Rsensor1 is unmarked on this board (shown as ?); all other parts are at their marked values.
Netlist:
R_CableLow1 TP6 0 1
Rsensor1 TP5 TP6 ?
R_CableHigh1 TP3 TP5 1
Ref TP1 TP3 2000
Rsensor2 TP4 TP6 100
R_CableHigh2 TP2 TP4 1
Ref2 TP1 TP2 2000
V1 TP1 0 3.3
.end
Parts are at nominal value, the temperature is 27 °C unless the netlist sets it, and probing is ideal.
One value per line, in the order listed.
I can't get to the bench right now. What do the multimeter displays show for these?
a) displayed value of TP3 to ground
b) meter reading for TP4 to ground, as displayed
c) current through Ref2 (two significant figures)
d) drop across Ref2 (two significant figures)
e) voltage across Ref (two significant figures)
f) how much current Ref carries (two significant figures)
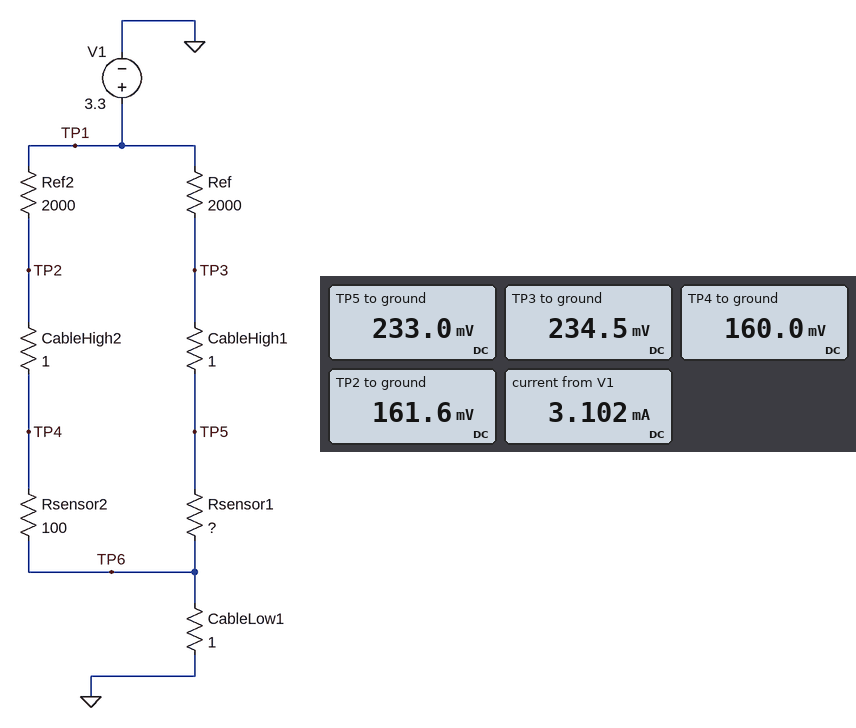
234.5 mV
160.0 mV
1.6 mA
3.1 V
3.1 V
1.5 mA
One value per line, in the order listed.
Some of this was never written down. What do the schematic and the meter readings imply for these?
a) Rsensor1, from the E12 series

150 Ω
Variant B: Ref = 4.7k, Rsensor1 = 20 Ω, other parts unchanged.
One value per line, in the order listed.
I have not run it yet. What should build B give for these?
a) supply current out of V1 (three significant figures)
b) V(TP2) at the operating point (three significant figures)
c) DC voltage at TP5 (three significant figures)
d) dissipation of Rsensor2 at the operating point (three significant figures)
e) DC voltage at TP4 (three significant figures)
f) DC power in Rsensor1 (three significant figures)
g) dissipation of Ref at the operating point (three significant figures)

2.27 mA
161 mV
16.2 mV
246 µW
159 mV
9.76 µW
2.29 mW
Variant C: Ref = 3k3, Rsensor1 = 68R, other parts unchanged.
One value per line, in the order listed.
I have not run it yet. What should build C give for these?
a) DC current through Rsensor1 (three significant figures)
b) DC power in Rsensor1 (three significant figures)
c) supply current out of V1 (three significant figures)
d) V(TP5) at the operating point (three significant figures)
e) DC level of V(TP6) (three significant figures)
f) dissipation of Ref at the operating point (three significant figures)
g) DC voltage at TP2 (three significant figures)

979 µA
65.1 µW
2.55 mA
69.1 mV
2.55 mV
3.16 mW
161 mV
